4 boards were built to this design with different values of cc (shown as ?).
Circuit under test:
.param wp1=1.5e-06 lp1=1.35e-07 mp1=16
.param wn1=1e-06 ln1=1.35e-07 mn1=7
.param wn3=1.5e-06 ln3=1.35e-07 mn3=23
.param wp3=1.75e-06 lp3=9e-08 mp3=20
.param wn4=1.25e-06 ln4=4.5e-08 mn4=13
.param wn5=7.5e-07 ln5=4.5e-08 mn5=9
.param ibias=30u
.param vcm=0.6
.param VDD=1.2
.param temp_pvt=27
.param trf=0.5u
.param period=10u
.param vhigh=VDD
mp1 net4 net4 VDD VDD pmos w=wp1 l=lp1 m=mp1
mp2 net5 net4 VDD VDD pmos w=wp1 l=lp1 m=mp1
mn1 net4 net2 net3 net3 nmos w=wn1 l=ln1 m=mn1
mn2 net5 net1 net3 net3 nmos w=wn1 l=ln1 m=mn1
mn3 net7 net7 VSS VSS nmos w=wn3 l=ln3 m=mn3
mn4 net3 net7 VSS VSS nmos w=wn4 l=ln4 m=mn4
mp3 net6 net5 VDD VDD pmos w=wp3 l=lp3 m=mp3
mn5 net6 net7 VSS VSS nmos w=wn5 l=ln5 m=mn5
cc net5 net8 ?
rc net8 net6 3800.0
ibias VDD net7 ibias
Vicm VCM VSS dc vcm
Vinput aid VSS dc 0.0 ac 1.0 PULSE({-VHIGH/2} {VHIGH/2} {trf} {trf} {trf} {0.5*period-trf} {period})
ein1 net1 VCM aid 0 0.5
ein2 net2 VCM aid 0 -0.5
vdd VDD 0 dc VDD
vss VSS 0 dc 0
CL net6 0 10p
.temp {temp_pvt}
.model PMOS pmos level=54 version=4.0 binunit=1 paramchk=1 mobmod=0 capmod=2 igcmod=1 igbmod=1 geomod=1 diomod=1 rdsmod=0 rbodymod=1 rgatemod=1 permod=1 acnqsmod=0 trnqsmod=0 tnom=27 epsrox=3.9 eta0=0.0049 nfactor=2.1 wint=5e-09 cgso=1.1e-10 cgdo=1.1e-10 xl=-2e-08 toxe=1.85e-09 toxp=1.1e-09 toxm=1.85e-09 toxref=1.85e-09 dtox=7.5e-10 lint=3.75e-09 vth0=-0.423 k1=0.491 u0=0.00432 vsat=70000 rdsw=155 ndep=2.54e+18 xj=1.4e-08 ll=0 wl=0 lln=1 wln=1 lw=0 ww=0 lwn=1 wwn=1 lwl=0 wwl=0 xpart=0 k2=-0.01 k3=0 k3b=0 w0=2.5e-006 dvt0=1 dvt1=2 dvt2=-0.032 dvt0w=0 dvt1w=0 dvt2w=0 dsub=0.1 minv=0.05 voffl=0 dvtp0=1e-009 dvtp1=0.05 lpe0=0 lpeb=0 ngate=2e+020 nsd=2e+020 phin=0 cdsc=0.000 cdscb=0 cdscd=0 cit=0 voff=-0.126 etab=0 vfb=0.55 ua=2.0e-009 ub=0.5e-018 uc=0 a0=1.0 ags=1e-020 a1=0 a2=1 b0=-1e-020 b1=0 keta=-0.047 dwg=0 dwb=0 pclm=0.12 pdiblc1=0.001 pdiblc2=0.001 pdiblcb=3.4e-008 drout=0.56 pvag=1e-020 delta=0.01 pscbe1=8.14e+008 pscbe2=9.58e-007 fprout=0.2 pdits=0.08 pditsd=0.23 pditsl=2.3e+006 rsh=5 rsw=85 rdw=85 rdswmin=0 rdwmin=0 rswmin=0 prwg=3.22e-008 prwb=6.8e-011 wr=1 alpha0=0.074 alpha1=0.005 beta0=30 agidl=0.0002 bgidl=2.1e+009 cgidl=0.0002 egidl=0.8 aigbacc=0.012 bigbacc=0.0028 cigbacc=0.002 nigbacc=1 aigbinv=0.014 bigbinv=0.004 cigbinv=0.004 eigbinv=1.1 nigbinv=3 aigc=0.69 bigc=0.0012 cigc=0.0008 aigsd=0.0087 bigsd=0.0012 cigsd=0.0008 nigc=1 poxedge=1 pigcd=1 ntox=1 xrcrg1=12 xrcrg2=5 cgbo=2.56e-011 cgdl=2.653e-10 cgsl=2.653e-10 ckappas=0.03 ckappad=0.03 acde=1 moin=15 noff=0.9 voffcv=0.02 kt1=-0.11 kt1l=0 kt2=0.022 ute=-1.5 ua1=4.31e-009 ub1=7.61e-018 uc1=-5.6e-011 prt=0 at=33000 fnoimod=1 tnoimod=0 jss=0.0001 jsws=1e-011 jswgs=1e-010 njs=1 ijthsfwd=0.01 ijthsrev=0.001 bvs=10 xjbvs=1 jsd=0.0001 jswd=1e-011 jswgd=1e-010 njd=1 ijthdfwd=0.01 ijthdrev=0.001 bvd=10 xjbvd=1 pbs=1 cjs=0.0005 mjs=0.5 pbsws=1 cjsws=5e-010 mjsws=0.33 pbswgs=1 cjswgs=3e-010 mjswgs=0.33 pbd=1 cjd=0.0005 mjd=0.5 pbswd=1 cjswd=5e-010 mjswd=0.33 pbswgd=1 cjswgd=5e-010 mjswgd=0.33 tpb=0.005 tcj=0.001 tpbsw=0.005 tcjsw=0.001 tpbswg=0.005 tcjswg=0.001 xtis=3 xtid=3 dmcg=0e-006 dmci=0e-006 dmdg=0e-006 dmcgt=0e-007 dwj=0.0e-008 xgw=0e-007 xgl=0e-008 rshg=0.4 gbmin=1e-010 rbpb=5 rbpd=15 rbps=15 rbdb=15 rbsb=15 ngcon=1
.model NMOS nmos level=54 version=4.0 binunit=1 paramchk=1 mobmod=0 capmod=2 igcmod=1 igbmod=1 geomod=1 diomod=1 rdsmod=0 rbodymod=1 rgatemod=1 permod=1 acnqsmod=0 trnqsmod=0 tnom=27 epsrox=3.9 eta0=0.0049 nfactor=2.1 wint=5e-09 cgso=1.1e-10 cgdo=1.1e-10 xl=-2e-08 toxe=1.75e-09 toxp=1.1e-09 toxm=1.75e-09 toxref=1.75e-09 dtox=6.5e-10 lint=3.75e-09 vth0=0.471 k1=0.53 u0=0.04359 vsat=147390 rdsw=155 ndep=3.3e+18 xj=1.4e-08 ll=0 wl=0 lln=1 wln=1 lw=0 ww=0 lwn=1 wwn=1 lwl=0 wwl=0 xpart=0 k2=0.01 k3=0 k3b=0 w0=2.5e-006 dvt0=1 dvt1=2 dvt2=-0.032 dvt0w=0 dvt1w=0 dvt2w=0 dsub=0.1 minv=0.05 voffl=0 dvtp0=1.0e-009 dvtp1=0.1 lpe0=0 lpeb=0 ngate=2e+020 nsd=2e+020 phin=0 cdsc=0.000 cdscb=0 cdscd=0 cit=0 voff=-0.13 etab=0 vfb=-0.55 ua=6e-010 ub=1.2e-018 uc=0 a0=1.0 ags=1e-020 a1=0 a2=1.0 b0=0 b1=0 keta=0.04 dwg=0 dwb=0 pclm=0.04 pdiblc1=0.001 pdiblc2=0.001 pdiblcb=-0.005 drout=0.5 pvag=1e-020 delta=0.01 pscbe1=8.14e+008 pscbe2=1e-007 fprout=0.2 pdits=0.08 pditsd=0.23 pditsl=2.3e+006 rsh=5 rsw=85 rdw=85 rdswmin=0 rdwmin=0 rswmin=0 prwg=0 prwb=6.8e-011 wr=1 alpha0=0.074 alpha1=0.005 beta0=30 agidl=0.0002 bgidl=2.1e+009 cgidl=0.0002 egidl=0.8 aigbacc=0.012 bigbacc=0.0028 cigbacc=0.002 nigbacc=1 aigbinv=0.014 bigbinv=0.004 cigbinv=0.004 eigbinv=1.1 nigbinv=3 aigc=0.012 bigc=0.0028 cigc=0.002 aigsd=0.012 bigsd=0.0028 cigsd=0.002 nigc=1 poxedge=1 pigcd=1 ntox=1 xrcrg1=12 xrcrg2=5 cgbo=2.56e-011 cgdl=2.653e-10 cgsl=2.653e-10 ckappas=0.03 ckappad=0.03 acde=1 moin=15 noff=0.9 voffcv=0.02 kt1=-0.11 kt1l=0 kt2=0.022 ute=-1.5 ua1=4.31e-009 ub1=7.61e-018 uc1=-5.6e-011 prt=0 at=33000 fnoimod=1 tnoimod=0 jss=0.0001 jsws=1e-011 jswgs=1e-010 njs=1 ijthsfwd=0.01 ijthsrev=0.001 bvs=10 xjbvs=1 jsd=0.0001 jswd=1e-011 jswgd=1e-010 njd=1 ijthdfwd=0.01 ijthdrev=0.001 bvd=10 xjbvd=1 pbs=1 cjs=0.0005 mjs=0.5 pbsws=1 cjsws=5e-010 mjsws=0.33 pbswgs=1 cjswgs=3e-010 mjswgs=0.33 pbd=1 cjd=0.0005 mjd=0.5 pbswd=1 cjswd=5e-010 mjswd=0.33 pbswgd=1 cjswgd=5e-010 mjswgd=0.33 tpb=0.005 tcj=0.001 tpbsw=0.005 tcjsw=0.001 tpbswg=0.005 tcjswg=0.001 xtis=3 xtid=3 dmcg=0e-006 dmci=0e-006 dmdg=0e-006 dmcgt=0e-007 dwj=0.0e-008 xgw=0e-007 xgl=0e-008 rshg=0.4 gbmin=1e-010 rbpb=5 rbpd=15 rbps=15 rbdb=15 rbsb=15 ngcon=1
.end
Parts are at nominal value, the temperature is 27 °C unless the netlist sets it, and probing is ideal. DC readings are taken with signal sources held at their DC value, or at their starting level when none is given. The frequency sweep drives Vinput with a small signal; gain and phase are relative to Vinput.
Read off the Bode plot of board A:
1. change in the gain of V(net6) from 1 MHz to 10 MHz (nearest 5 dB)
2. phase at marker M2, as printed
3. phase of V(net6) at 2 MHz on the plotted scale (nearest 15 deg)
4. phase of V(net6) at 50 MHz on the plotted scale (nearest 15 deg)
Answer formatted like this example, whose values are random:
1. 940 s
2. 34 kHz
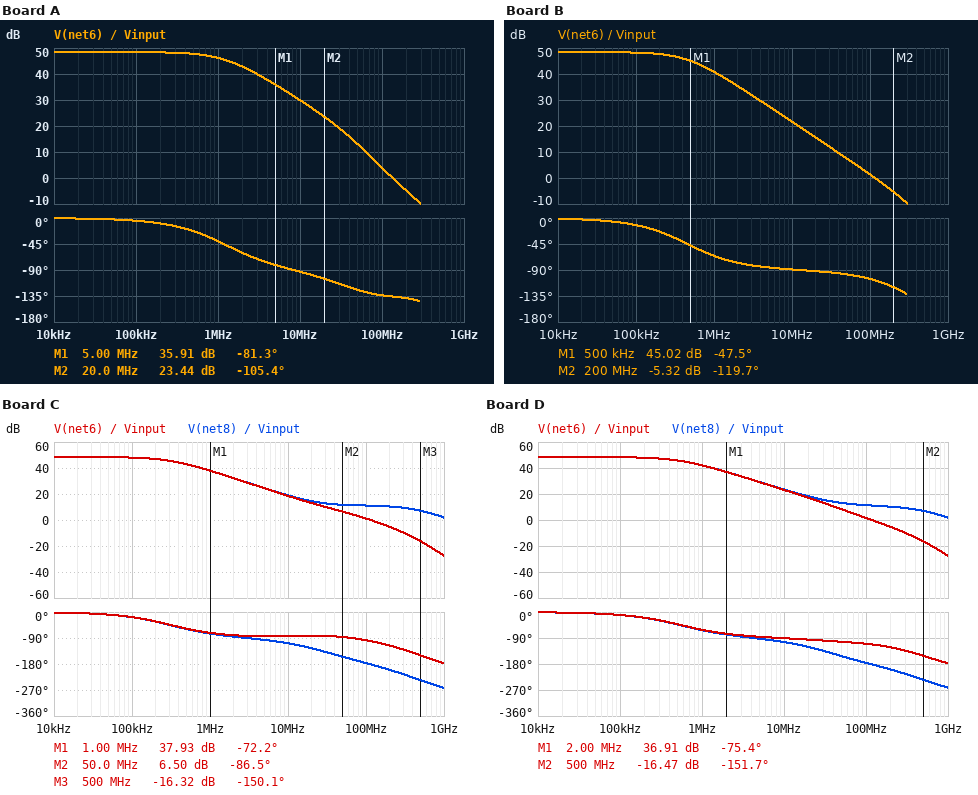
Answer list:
1. -15 dB
2. -105.4 deg
3. -60 deg
4. -120 deg
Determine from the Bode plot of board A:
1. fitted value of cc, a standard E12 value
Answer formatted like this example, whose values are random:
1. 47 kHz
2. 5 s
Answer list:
1. 330 fF
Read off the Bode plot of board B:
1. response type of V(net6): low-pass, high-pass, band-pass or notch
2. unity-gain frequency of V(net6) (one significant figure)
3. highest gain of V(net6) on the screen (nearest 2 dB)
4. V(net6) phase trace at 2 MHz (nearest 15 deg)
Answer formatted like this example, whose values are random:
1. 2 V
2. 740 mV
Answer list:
1. low-pass
2. 100 MHz
3. 48 dB
4. -75 deg
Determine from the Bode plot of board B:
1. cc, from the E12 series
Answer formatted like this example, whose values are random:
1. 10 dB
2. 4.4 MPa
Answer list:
1. 1 pF
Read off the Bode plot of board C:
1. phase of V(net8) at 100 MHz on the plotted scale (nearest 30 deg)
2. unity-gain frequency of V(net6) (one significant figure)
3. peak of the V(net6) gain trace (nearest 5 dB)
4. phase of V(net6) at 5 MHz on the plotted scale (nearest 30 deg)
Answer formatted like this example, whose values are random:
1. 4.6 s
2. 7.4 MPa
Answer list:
1. -180 deg
2. 100 MHz
3. 50 dB
4. -90 deg
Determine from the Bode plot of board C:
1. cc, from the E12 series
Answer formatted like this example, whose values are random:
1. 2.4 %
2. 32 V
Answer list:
1. 1.5 pF
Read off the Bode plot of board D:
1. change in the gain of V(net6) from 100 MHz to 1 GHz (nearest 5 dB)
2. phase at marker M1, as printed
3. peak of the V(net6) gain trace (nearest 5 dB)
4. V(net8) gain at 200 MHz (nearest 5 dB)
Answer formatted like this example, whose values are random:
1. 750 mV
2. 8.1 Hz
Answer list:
1. -30 dB
2. -75.4 deg
3. 50 dB
4. 10 dB
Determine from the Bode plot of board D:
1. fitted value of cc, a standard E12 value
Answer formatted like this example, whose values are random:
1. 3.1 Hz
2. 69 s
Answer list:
1. 820 fF
